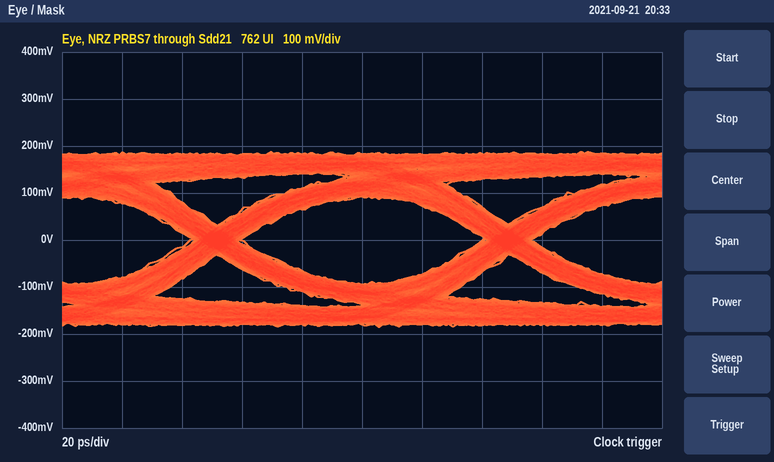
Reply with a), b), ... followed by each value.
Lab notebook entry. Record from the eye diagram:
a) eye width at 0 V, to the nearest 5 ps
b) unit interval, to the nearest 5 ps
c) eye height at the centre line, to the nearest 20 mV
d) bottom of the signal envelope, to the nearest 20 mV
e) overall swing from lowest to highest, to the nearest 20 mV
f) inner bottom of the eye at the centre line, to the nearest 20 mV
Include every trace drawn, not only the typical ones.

a) 80 ps
b) 95 ps
c) 180 mV
d) -180 mV
e) 380 mV
f) -100 mV
